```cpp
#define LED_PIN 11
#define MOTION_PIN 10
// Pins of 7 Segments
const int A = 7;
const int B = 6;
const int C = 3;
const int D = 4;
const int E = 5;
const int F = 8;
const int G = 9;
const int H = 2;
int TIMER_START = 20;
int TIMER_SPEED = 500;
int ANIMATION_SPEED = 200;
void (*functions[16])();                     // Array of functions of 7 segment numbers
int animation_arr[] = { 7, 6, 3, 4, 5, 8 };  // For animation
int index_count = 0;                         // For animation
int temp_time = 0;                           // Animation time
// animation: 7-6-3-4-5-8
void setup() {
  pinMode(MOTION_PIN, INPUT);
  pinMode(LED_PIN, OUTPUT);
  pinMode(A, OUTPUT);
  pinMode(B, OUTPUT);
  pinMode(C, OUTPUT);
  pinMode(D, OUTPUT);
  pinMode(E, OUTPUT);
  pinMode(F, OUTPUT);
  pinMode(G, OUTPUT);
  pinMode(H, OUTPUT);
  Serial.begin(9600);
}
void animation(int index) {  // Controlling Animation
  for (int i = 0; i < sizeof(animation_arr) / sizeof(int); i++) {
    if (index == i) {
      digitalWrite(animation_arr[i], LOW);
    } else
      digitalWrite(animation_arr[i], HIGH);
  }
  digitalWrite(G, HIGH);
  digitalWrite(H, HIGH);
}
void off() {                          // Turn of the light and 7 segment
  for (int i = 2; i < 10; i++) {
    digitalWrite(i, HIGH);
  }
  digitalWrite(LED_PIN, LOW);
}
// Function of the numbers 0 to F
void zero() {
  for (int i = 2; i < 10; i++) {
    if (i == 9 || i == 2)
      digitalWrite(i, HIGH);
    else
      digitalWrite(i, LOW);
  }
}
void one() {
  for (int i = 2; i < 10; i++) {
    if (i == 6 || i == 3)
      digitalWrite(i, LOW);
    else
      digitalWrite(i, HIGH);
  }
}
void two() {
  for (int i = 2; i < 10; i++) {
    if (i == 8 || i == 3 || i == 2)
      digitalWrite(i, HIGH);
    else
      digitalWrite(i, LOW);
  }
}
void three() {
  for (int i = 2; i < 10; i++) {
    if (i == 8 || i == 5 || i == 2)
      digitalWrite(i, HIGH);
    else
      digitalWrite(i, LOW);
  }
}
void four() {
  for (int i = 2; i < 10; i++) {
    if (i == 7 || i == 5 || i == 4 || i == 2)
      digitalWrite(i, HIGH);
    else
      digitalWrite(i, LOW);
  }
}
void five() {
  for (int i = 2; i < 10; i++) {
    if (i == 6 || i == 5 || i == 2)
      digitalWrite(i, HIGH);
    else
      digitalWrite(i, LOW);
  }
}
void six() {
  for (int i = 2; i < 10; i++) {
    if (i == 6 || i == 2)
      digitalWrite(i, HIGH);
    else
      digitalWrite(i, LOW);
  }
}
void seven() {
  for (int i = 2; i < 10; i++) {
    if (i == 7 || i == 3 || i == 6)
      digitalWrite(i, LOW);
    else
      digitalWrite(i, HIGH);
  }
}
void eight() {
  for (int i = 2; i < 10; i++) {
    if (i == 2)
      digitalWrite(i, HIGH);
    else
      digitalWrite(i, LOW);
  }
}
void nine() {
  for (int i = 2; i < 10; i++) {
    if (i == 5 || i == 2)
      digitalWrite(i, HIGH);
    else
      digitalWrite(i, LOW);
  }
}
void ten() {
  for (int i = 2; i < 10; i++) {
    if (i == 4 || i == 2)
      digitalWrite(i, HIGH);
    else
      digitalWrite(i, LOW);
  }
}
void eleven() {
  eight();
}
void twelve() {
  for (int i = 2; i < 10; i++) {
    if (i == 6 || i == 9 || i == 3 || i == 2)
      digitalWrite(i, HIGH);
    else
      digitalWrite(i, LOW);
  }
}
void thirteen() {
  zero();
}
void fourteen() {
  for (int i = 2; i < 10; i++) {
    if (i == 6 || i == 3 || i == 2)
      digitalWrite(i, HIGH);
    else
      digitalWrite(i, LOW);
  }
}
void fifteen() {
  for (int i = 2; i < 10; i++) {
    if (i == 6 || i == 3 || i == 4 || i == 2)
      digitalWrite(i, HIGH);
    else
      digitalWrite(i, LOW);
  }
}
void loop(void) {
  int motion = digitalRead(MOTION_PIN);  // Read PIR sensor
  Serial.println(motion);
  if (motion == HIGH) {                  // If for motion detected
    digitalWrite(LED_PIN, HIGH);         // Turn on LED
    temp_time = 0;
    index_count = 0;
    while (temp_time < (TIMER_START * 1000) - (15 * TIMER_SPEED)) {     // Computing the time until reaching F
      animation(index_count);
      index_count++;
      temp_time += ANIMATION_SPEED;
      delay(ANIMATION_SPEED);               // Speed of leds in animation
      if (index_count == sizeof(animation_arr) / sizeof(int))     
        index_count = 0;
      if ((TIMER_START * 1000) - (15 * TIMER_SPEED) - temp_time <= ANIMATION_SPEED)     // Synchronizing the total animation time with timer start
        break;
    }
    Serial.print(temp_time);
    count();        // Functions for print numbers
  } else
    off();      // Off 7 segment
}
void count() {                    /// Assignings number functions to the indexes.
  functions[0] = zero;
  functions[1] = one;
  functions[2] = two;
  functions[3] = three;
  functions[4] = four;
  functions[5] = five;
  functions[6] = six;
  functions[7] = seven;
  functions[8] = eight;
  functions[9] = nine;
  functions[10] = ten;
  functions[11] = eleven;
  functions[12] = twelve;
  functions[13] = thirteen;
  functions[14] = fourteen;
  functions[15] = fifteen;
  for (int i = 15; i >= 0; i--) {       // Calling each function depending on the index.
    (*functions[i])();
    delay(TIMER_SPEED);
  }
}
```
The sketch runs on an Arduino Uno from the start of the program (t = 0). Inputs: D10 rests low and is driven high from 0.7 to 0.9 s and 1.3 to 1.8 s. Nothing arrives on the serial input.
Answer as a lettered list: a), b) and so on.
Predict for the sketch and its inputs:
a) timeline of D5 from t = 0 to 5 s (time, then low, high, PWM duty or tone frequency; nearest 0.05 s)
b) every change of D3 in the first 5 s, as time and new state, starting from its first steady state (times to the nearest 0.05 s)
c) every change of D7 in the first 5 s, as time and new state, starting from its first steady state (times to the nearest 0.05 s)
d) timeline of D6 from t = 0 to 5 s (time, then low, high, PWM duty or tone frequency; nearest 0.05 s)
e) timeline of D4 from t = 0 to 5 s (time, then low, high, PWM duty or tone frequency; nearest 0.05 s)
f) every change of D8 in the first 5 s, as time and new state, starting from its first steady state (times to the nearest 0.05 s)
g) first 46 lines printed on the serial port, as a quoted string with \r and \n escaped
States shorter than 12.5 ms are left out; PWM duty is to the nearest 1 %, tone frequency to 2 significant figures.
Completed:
a) 0 s high; 1.5 s low; 1.7 s high; 2.7 s low; 2.9 s high; 3.9 s low; 4.1 s high
b) 0 s high; 1.1 s low; 1.3 s high; 2.3 s low; 2.5 s high; 3.5 s low; 3.7 s high; 4.7 s low; 4.9 s high
c) 0 s high; 0.7 s low; 0.9 s high; 1.9 s low; 2.1 s high; 3.1 s low; 3.3 s high; 4.3 s low; 4.5 s high
d) 0 s high; 0.9 s low; 1.1 s high; 2.1 s low; 2.3 s high; 3.3 s low; 3.5 s high; 4.5 s low; 4.7 s high
e) 0 s high; 1.3 s low; 1.5 s high; 2.5 s low; 2.7 s high; 3.7 s low; 3.9 s high; 4.9 s low
f) 0 s high; 1.7 s low; 1.9 s high; 2.9 s low; 3.1 s high; 4.1 s low; 4.3 s high
g) "0\r\n0\r\n0\r\n0\r\n0\r\n0\r\n0\r\n0\r\n0\r\n0\r\n0\r\n0\r\n0\r\n0\r\n0\r\n0\r\n0\r\n0\r\n0\r\n0\r\n0\r\n0\r\n0\r\n0\r\n0\r\n0\r\n0\r\n0\r\n0\r\n0\r\n0\r\n0\r\n0\r\n0\r\n0\r\n0\r\n0\r\n0\r\n0\r\n0\r\n0\r\n0\r\n0\r\n0\r\n0\r\n0\r\n"
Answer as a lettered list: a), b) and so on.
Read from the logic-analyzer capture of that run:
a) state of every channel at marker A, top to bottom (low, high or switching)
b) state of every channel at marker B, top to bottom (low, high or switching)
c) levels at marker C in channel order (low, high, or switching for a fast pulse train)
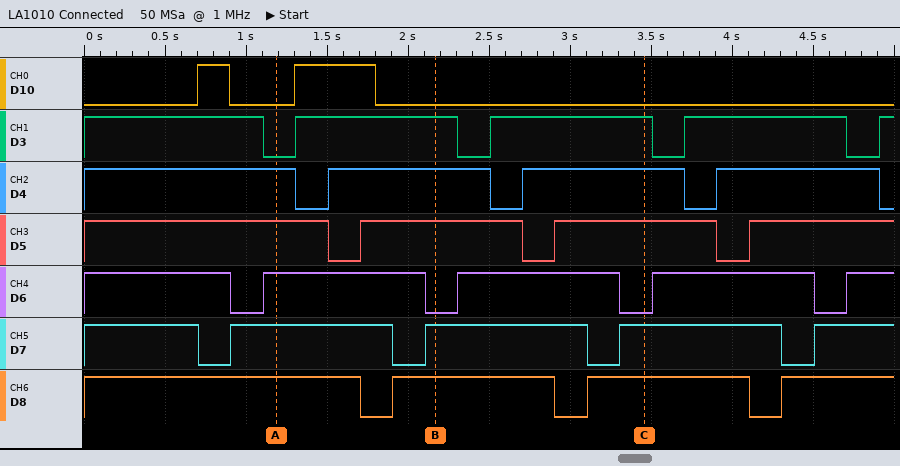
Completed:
a) D10 low, D3 low, D4 high, D5 high, D6 high, D7 high, D8 high
b) D10 low, D3 high, D4 high, D5 high, D6 low, D7 high, D8 high
c) D10 low, D3 high, D4 high, D5 high, D6 low, D7 high, D8 high
